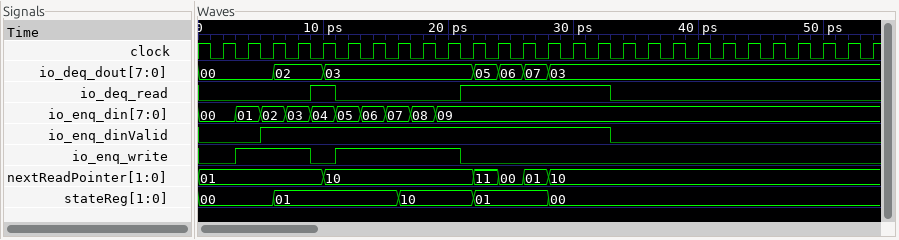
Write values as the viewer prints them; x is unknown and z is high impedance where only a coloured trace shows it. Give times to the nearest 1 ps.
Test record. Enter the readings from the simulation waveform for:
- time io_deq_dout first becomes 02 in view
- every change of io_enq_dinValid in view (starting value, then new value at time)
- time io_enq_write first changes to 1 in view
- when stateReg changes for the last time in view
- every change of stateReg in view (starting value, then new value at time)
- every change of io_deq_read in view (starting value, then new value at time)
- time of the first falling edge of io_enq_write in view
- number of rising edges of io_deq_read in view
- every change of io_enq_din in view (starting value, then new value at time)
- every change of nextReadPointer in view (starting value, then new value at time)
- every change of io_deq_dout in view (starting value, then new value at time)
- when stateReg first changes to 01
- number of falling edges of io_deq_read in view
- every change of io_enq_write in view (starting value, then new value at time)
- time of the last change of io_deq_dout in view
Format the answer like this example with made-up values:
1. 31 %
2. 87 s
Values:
1. 6 ps
2. 0, 1 at 5 ps, 0 at 33 ps
3. 3 ps
4. 28 ps
5. 00, 01 at 6 ps, 10 at 16 ps, 01 at 22 ps, 00 at 28 ps
6. 0, 1 at 9 ps, 0 at 11 ps, 1 at 21 ps, 0 at 33 ps
7. 9 ps
8. 2
9. 00, 01 at 3 ps, 02 at 5 ps, 03 at 7 ps, 04 at 9 ps, 05 at 11 ps, 06 at 13 ps, 07 at 15 ps, 08 at 17 ps, 09 at 19 ps
10. 01, 10 at 10 ps, 11 at 22 ps, 00 at 24 ps, 01 at 26 ps, 10 at 28 ps
11. 00, 02 at 6 ps, 03 at 10 ps, 05 at 22 ps, 06 at 24 ps, 07 at 26 ps, 03 at 28 ps
12. 6 ps
13. 2
14. 0, 1 at 3 ps, 0 at 9 ps, 1 at 11 ps, 0 at 21 ps
15. 28 ps
